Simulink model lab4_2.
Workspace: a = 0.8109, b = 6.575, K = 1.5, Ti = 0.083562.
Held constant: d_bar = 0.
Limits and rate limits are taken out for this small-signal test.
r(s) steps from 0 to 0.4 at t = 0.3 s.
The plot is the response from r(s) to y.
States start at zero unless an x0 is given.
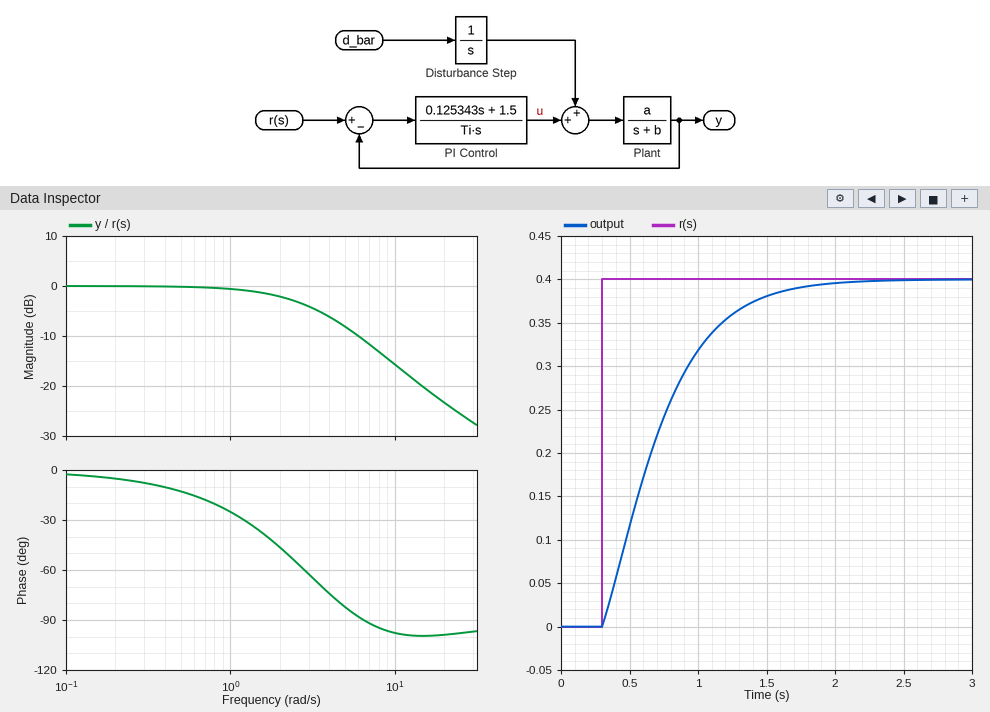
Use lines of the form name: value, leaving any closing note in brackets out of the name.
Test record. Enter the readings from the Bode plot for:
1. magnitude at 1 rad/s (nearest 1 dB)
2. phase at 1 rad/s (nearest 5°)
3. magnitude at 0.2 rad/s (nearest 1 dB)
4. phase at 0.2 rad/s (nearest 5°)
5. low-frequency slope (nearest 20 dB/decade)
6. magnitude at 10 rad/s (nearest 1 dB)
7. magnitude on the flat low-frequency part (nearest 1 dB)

magnitude at 1 rad/s: -1 dB
phase at 1 rad/s: -25°
magnitude at 0.2 rad/s: 0 dB
phase at 0.2 rad/s: -5°
low-frequency slope: 0 dB/decade
magnitude at 10 rad/s: -16 dB
magnitude on the flat low-frequency part: 0 dB
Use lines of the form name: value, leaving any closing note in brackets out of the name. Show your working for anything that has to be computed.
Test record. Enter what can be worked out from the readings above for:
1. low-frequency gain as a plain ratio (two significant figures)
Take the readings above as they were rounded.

low-frequency gain as a plain ratio: 10^(0 / 20) = 1.0
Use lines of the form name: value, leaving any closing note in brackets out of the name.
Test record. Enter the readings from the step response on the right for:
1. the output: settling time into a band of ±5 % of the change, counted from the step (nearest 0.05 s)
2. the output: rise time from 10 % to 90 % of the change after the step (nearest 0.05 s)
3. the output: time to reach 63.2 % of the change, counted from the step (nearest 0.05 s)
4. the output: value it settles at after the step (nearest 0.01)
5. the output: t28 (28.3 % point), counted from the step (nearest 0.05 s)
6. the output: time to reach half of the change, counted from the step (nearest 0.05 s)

the output: settling time into a band of ±5 % of the change, counted from the step: 1.20 s
the output: rise time from 10 % to 90 % of the change after the step: 0.90 s
the output: time to reach 63.2 % of the change, counted from the step: 0.50 s
the output: value it settles at after the step: 0.40
the output: t28 (28.3 % point), counted from the step: 0.20 s
the output: time to reach half of the change, counted from the step: 0.35 s
